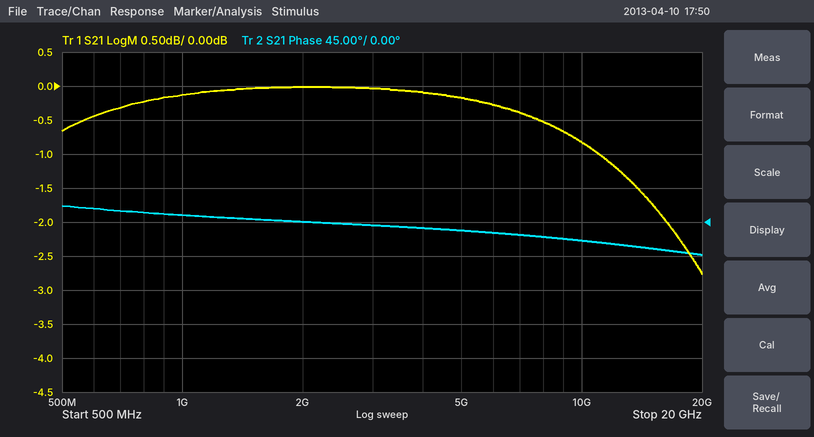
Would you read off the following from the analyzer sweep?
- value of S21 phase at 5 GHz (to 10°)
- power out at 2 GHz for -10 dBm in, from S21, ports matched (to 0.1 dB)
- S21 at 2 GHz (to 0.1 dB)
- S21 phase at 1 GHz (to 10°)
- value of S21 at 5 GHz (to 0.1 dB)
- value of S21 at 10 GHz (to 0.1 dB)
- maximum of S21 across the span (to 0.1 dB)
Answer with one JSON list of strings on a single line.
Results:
["-10°", "-10.0 dBm", "0.0 dB", "10°", "-0.2 dB", "-0.8 dB", "0.0 dB"]
